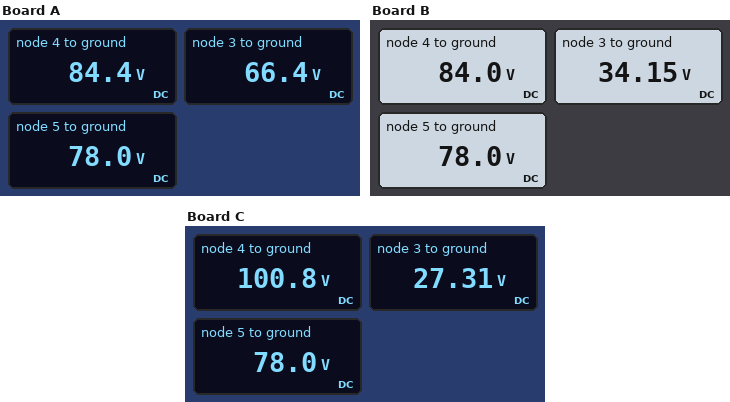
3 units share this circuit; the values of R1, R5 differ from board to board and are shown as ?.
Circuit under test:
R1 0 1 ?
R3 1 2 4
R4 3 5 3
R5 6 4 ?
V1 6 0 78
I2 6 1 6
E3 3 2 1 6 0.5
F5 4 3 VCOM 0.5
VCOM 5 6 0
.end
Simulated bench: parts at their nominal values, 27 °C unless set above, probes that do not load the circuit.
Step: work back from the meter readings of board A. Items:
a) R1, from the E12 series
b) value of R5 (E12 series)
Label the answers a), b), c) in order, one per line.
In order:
a) 8.2 Ω
b) 3.3 Ω
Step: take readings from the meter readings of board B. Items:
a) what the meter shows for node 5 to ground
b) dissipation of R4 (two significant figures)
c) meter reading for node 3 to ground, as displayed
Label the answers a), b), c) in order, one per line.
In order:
a) 78.0 V
b) 640 W
c) 34.15 V
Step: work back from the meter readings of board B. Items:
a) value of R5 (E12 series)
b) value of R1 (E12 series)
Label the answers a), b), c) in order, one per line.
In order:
a) 0.82 Ω
b) 2.2 Ω
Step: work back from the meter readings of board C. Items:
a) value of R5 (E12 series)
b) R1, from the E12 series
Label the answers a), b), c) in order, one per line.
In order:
a) 2.7 Ω
b) 1.5 Ω
